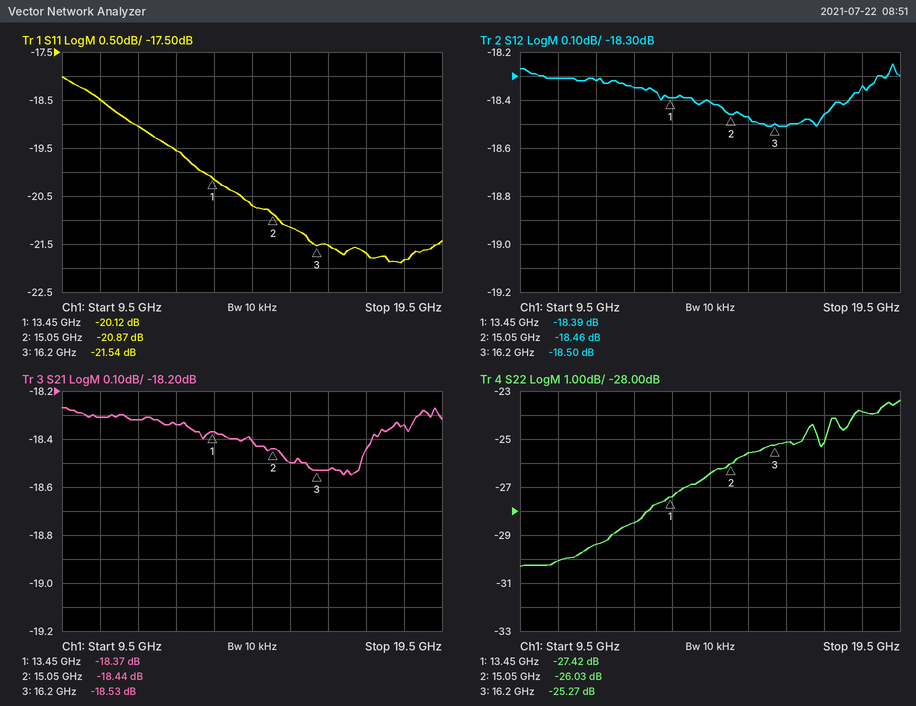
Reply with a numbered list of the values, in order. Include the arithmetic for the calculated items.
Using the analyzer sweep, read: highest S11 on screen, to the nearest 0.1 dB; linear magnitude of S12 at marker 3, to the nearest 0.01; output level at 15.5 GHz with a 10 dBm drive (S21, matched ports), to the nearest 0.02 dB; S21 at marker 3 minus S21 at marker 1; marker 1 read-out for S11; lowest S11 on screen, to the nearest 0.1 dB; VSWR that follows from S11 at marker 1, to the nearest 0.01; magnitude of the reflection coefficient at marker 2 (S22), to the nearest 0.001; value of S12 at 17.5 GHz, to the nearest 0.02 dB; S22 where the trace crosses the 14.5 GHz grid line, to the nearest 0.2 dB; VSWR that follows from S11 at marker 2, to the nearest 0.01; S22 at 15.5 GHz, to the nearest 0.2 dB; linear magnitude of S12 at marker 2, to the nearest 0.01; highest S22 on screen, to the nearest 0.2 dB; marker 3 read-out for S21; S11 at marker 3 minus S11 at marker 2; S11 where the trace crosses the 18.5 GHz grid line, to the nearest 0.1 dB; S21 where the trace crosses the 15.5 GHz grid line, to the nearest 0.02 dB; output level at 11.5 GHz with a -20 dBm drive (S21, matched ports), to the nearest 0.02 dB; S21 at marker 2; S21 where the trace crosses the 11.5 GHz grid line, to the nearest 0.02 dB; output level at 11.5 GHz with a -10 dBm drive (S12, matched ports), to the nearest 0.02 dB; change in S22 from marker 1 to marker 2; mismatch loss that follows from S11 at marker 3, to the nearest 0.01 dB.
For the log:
1. -18.0 dB
2. 10^(-18.5/20) ≈ 0.12
3. 10 dBm + (-18.50 dB) = -8.50 dBm
4. -18.53 − (-18.37) = -0.16 dB
5. -20.12 dB
6. -21.9 dB
7. (1 + 0.0986)/(1 − 0.0986) ≈ 1.22
8. 10^(-26.03/20) ≈ 0.050
9. -18.46 dB
10. -26.4 dB
11. (1 + 0.0905)/(1 − 0.0905) ≈ 1.20
12. -25.6 dB
13. 10^(-18.46/20) ≈ 0.12
14. -23.4 dB
15. -18.53 dB
16. -21.54 − (-20.87) = -0.67 dB
17. -21.8 dB
18. -18.50 dB
19. -20 dBm + (-18.32 dB) = -38.32 dBm
20. -18.44 dB
21. -18.32 dB
22. -10 dBm + (-18.32 dB) = -28.32 dBm
23. -26.03 − (-27.42) = 1.39 dB
24. −10 log10(1 − 10^(-21.54/10)) ≈ 0.03 dB
